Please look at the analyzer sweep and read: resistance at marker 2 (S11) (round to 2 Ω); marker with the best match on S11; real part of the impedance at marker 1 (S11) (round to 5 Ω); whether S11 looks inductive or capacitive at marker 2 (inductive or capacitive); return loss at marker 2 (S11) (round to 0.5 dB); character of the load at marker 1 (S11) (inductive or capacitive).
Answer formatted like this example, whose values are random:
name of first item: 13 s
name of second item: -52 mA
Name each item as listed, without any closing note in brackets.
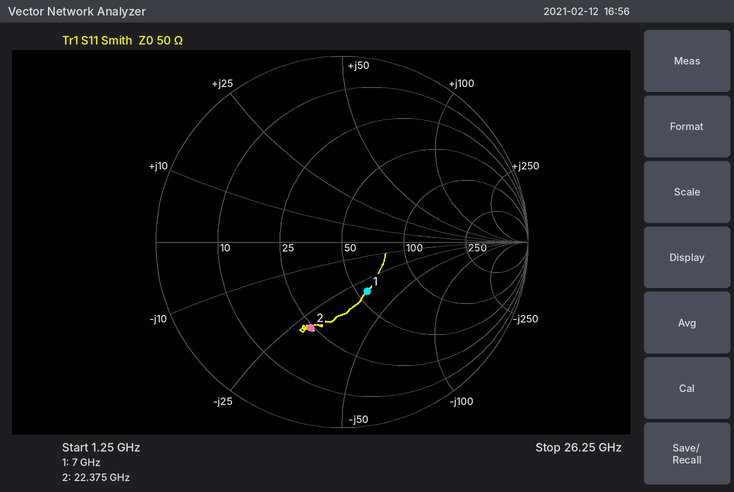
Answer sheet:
resistance at marker 2 (S11): 24 Ω
marker with the best match on S11: marker 1
real part of the impedance at marker 1 (S11): 55 Ω
whether S11 looks inductive or capacitive at marker 2: capacitive
return loss at marker 2 (S11): 6.0 dB
character of the load at marker 1 (S11): capacitive
